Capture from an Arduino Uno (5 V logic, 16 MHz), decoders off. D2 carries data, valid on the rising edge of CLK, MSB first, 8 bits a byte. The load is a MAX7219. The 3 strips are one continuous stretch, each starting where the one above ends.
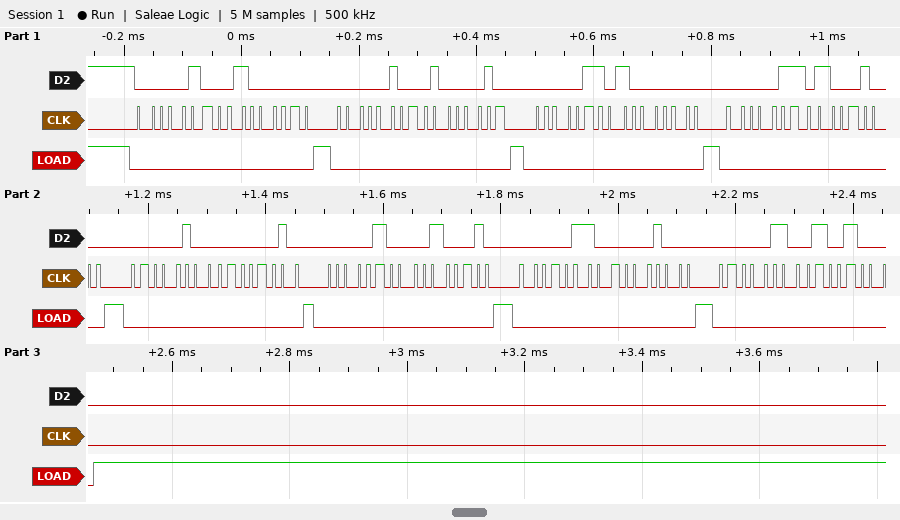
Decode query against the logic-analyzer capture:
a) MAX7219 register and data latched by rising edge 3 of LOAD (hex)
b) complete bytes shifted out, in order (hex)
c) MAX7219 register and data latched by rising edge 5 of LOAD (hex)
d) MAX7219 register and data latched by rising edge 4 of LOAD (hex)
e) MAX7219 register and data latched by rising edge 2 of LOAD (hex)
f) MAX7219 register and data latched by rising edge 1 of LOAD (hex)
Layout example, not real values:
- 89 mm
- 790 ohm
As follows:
- register 0x6, data 0x80
- 04 40 04 42 06 80 06 88 04 02 04 22 06 08 06 48
- register 0x4, data 0x02
- register 0x6, data 0x88
- register 0x4, data 0x42
- register 0x4, data 0x40
